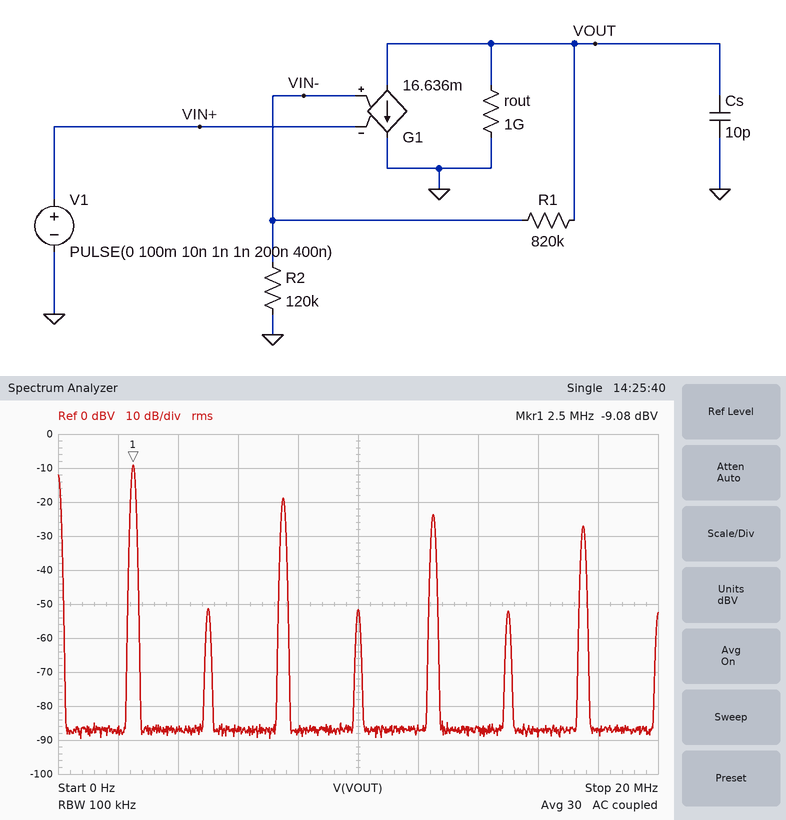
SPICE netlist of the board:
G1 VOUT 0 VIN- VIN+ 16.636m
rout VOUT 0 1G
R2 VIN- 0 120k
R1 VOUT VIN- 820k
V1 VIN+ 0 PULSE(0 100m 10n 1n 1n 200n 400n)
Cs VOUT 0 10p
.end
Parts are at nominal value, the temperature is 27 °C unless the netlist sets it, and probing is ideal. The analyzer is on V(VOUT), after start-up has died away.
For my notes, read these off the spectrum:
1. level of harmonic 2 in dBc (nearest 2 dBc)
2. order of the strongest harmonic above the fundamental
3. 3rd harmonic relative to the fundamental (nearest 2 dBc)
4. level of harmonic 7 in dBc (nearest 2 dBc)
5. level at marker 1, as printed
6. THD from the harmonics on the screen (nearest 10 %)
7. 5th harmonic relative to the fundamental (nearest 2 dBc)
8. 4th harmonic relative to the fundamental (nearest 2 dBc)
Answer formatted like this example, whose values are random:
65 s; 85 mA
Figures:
-42 dBc; 3; -10 dBc; -18 dBc; -9.08 dBV; 40 %; -14 dBc; -42 dBc
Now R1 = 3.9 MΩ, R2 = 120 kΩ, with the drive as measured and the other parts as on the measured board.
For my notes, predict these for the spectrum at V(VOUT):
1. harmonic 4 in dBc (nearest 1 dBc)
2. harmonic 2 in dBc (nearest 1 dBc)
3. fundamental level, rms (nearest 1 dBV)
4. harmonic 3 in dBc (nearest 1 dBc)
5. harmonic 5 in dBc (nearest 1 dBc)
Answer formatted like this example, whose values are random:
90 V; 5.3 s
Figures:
-46 dBc; -43 dBc; 3 dBV; -12 dBc; -19 dBc
